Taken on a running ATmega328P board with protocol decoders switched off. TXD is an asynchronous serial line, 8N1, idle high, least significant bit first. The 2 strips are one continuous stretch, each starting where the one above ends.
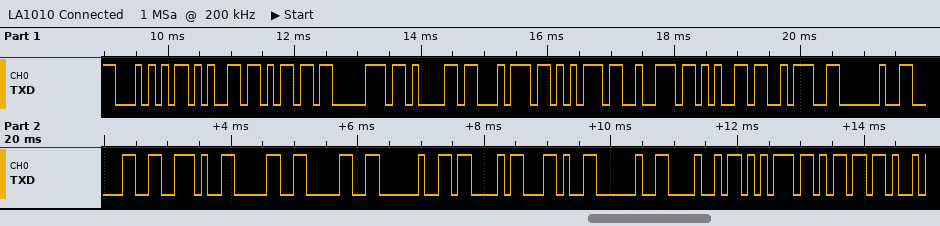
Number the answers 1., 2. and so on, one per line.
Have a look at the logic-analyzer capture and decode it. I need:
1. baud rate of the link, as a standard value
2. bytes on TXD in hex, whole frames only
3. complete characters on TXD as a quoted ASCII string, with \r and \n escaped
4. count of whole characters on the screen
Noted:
1. 9600 baud
2. 0x54 0x65 0x6D 0x70 0x61 0x74 0x75 0x72 0x65 0x3A 0x20 0x30 0x2E 0x30 0x30 0x20 0x43 0x2C 0x20 0x48 0x75 0x6D
3. "Tempature: 0.00 C, Hum"
4. 22
